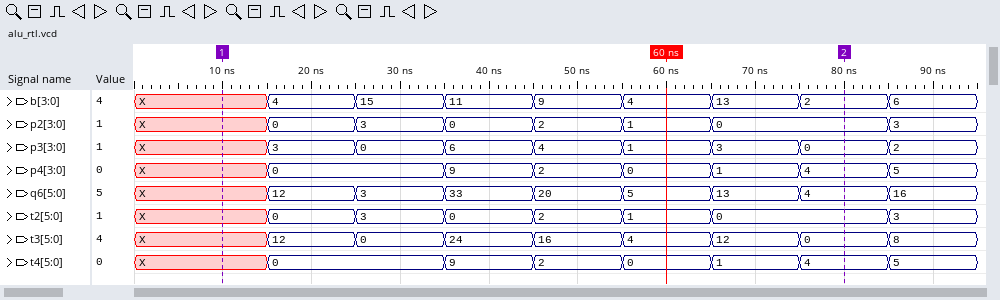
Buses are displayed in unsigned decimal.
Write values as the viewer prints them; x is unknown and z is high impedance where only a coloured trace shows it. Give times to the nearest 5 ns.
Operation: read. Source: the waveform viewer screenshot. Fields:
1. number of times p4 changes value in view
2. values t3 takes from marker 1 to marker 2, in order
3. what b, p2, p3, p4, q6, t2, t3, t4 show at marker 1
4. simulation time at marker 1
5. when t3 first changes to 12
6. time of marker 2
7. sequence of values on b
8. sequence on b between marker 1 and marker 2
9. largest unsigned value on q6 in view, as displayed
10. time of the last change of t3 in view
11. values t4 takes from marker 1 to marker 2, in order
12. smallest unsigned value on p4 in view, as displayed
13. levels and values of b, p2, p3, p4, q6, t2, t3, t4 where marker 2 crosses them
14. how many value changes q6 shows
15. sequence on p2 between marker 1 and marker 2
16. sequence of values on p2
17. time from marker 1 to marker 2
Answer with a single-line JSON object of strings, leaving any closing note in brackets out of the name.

{"number of times p4 changes value in view": "7", "values t3 takes from marker 1 to marker 2, in order": "X, 12, 0, 24, 16, 4, 12, 0", "what b, p2, p3, p4, q6, t2, t3, t4 show at marker 1": "b=X, p2=X, p3=X, p4=X, q6=X, t2=X, t3=X, t4=X", "simulation time at marker 1": "10 ns", "when t3 first changes to 12": "15 ns", "time of marker 2": "80 ns", "sequence of values on b": "X, 4, 15, 11, 9, 4, 13, 2, 6", "sequence on b between marker 1 and marker 2": "X, 4, 15, 11, 9, 4, 13, 2", "largest unsigned value on q6 in view, as displayed": "33", "time of the last change of t3 in view": "85 ns", "values t4 takes from marker 1 to marker 2, in order": "X, 0, 9, 2, 0, 1, 4", "smallest unsigned value on p4 in view, as displayed": "0", "levels and values of b, p2, p3, p4, q6, t2, t3, t4 where marker 2 crosses them": "b=2, p2=0, p3=0, p4=4, q6=4, t2=0, t3=0, t4=4", "how many value changes q6 shows": "8", "sequence on p2 between marker 1 and marker 2": "X, 0, 3, 0, 2, 1, 0", "sequence of values on p2": "X, 0, 3, 0, 2, 1, 0, 3", "time from marker 1 to marker 2": "70 ns"}
